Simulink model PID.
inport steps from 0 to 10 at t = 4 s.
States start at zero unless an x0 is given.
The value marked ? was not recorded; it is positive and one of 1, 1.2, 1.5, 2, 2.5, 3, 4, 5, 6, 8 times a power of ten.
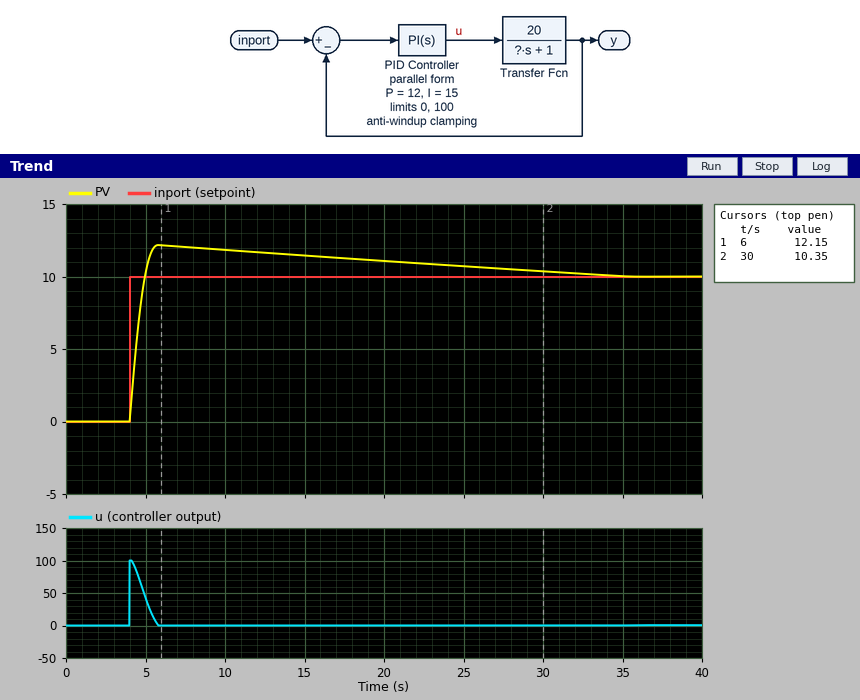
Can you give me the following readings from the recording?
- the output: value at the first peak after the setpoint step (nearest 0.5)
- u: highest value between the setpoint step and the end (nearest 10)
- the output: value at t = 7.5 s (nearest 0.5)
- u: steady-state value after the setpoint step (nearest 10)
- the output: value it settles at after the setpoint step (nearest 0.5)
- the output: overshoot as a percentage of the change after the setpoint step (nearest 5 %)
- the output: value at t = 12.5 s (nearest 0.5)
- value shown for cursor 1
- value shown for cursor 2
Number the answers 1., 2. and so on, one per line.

1. 12.0
2. 100
3. 12.0
4. 0
5. 10.0
6. 20 %
7. 11.5
8. 12.15
9. 10.35
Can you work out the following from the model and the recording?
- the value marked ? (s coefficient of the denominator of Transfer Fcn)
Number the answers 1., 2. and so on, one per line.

1. 150
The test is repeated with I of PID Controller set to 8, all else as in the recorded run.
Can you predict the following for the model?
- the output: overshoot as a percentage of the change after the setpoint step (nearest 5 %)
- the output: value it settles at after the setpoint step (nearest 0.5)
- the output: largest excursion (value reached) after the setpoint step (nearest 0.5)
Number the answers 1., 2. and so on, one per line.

1. 15 %
2. 10.0
3. 11.5
